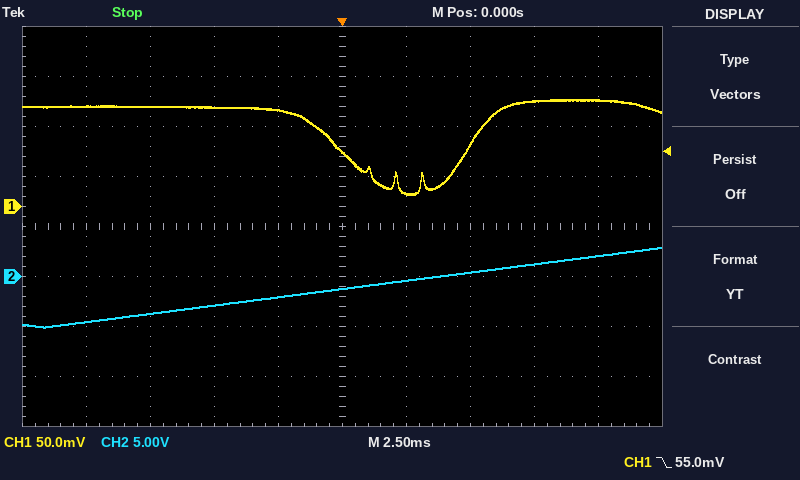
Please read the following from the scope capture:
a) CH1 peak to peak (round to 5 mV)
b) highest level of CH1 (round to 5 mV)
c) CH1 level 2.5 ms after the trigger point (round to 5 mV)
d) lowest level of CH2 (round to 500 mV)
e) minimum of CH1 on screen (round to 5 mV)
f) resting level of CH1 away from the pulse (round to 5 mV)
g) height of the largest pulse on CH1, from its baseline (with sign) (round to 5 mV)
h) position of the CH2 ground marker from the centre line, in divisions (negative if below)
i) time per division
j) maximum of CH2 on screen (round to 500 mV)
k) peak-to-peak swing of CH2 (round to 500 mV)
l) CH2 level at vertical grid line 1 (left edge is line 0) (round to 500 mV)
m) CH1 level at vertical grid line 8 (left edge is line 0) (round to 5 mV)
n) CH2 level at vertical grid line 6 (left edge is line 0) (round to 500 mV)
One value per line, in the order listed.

95 mV
105 mV
15 mV
-5.0 V
10 mV
100 mV
-90 mV
-1.0 div
2.5 ms
3.0 V
8.0 V
-4.5 V
105 mV
-500 mV
